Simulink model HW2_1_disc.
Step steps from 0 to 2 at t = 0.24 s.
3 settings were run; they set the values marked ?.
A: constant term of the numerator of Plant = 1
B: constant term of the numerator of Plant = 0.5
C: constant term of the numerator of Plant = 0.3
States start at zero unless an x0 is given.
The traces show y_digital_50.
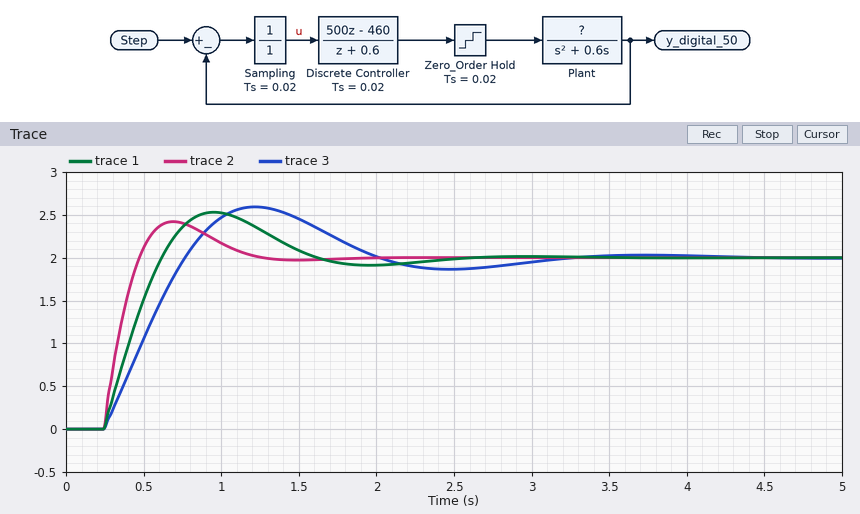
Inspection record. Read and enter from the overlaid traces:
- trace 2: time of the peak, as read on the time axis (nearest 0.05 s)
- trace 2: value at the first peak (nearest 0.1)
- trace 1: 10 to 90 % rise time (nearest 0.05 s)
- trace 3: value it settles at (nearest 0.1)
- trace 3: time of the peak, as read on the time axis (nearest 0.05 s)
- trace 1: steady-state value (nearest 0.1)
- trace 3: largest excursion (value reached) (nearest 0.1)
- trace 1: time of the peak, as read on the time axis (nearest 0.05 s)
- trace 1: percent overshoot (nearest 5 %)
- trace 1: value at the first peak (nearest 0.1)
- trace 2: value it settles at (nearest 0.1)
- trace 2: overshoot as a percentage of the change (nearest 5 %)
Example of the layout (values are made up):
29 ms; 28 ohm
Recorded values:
0.70 s; 2.4; 0.30 s; 2.0; 1.20 s; 2.0; 2.6; 0.95 s; 25 %; 2.5; 2.0; 20 %
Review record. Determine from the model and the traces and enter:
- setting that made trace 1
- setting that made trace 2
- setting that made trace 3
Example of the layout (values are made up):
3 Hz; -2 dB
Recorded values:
B; A; C
